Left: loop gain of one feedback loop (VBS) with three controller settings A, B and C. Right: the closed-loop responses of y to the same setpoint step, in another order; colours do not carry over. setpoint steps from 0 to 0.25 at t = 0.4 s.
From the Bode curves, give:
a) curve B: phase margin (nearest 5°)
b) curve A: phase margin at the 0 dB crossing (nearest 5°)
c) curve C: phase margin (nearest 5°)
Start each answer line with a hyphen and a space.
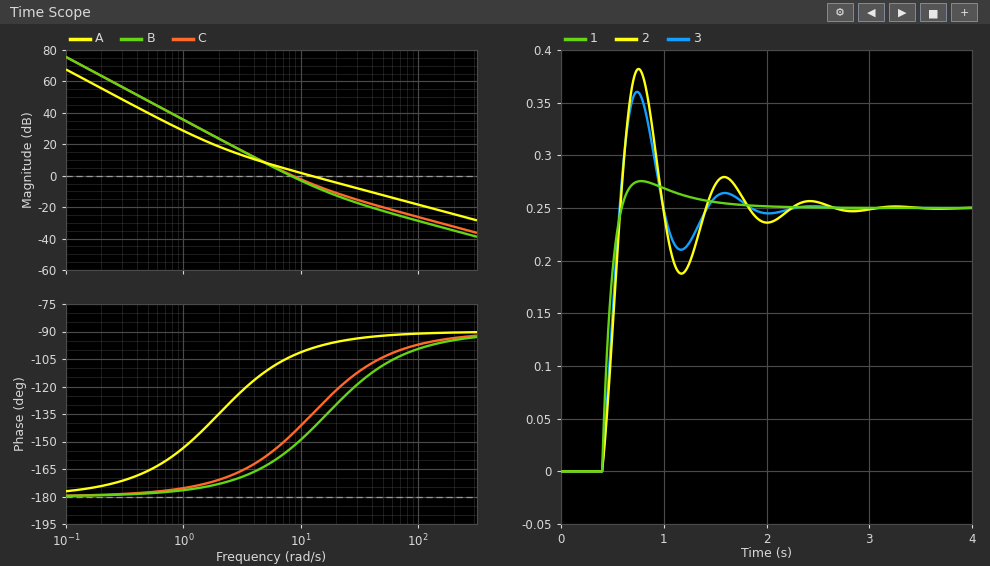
- 25°
- 80°
- 35°
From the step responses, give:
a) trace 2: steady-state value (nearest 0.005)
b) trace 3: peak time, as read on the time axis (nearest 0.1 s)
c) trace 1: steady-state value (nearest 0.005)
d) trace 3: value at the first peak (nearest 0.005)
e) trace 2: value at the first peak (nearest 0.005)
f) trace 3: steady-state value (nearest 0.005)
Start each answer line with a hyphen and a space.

- 0.250
- 0.7 s
- 0.250
- 0.360
- 0.380
- 0.250
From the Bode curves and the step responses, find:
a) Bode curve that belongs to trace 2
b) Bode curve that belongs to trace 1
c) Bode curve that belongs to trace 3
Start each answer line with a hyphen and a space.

- B
- A
- C
